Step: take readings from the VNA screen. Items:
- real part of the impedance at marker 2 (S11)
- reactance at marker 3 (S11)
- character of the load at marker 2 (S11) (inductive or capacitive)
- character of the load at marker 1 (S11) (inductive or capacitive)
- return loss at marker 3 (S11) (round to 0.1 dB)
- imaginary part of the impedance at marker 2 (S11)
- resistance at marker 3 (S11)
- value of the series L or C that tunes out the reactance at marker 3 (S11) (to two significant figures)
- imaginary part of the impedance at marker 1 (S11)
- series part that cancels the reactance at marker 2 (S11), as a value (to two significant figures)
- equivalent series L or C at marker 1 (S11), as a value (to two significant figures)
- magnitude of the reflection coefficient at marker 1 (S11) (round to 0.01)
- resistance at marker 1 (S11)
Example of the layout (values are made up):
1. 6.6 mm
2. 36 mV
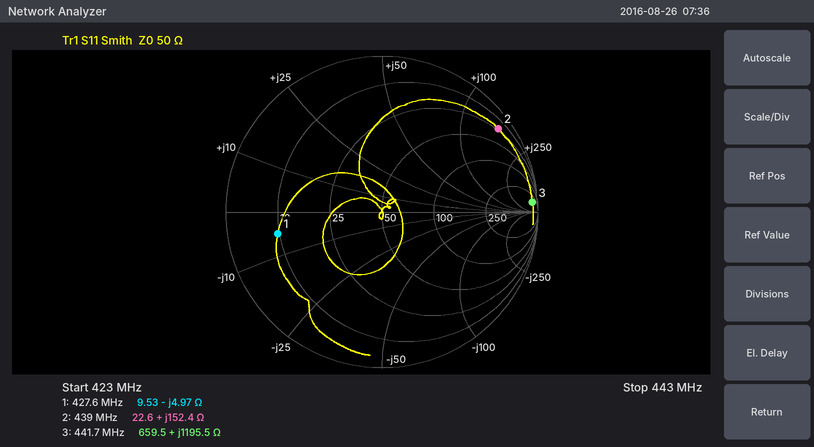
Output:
1. 22.6 Ω
2. +1195.5 Ω
3. inductive
4. capacitive
5. 0.3 dB
6. +152.4 Ω
7. 659.5 Ω
8. 300 fF
9. -4.97 Ω
10. 2.4 pF
11. 75 pF
12. 0.68
13. 9.53 Ω
